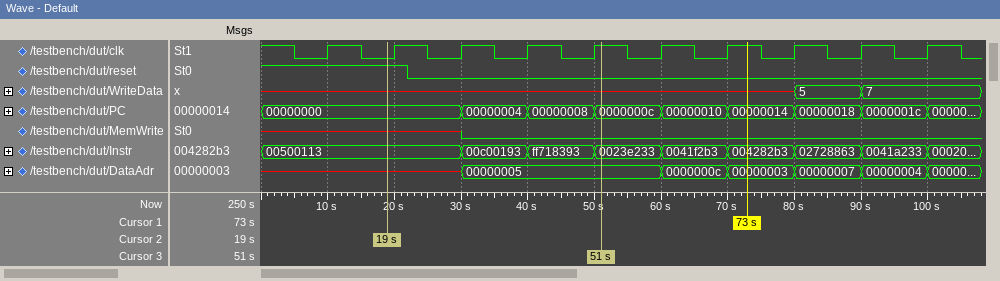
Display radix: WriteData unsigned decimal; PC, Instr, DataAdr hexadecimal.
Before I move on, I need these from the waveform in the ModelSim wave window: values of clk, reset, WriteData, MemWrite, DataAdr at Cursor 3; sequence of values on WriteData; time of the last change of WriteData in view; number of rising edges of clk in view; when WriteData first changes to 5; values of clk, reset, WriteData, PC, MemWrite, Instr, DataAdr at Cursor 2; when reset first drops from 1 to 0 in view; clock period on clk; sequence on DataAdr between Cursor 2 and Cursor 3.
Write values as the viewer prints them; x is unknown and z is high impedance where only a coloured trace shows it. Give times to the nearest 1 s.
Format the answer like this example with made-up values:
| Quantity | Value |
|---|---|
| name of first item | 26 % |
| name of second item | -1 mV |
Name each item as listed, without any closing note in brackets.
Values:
| Quantity | Value |
|---|---|
| values of clk, reset, WriteData, MemWrite, DataAdr at Cursor 3 | clk=1, reset=0, WriteData=x, MemWrite=0, DataAdr=00000005 |
| sequence of values on WriteData | x, 5, 7 |
| time of the last change of WriteData in view | 90 s |
| number of rising edges of clk in view | 10 |
| when WriteData first changes to 5 | 80 s |
| values of clk, reset, WriteData, PC, MemWrite, Instr, DataAdr at Cursor 2 | clk=0, reset=1, WriteData=x, PC=00000000, MemWrite=x, Instr=00500113, DataAdr=x |
| when reset first drops from 1 to 0 in view | 22 s |
| clock period on clk | 10 s |
| sequence on DataAdr between Cursor 2 and Cursor 3 | x, 00000005 |
